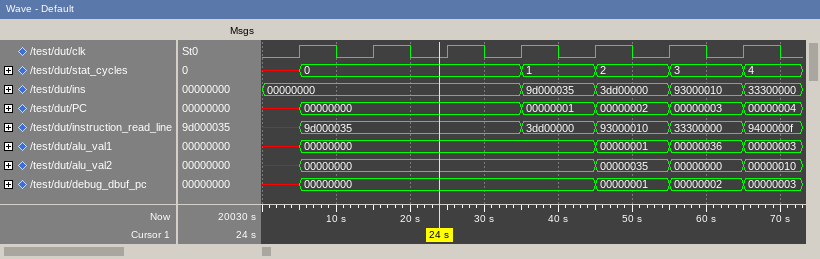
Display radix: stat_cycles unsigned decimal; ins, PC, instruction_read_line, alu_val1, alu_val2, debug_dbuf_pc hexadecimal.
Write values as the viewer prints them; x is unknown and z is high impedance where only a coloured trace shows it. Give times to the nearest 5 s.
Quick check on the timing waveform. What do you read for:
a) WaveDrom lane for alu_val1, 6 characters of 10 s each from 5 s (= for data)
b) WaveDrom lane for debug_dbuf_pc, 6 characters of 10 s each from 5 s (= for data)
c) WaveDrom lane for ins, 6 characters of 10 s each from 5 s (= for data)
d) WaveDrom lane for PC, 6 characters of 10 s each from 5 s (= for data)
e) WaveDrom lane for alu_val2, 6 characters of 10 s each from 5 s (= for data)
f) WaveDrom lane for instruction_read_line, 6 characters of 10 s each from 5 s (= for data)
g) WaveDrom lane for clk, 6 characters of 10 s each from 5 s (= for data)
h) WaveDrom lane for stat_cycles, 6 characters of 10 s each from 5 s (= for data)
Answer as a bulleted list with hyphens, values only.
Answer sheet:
- {name: 'alu_val1', wave: '=...==', data: '00000000 00000001 00000036'}
- {name: 'debug_dbuf_pc', wave: '=...==', data: '00000000 00000001 00000002'}
- {name: 'ins', wave: '=..===', data: '00000000 9d000035 3dd00000 93000010'}
- {name: 'PC', wave: '=..===', data: '00000000 00000001 00000002 00000003'}
- {name: 'alu_val2', wave: '=...==', data: '00000000 00000035 00000000'}
- {name: 'instruction_read_line', wave: '=..===', data: '9d000035 3dd00000 93000010 33300000'}
- {name: 'clk', wave: 'p.....'}
- {name: 'stat_cycles', wave: '=..===', data: '0 1 2 3'}
